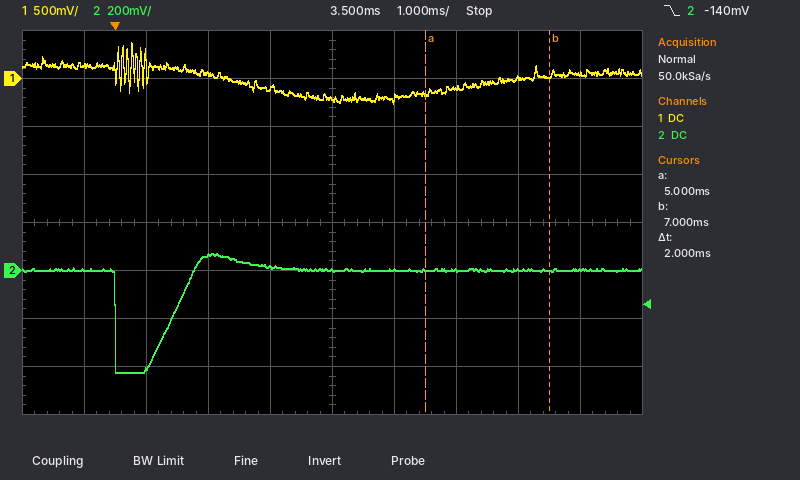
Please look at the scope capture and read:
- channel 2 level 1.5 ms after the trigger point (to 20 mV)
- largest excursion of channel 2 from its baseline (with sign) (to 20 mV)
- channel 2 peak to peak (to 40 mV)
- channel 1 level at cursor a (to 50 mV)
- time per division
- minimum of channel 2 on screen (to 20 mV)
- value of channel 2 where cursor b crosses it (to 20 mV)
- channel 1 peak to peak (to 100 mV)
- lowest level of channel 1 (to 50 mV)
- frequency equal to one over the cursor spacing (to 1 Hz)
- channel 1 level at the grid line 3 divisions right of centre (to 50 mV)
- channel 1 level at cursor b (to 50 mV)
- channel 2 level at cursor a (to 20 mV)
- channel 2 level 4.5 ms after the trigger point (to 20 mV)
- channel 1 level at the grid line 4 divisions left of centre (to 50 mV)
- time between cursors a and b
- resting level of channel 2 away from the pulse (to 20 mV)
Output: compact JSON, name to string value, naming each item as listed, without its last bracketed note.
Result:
{"channel 2 level 1.5 ms after the trigger point": "60 mV", "largest excursion of channel 2 from its baseline (with sign)": "-420 mV", "channel 2 peak to peak": "480 mV", "channel 1 level at cursor a": "-150 mV", "time per division": "1 ms", "minimum of channel 2 on screen": "-420 mV", "value of channel 2 where cursor b crosses it": "0 mV", "channel 1 peak to peak": "600 mV", "lowest level of channel 1": "-250 mV", "frequency equal to one over the cursor spacing": "500 Hz", "channel 1 level at the grid line 3 divisions right of centre": "0 mV", "channel 1 level at cursor b": "50 mV", "channel 2 level at cursor a": "0 mV", "channel 2 level 4.5 ms after the trigger point": "0 mV", "channel 1 level at the grid line 4 divisions left of centre": "150 mV", "time between cursors a and b": "2 ms", "resting level of channel 2 away from the pulse": "0 mV"}
